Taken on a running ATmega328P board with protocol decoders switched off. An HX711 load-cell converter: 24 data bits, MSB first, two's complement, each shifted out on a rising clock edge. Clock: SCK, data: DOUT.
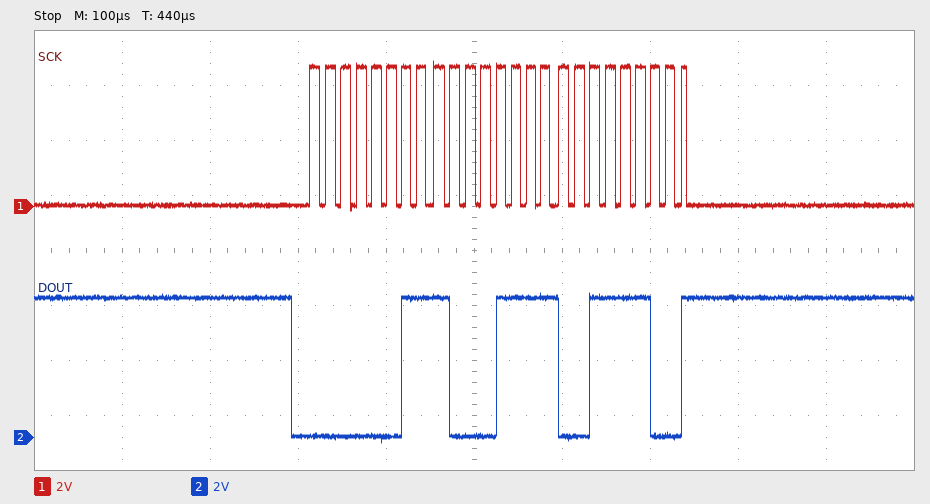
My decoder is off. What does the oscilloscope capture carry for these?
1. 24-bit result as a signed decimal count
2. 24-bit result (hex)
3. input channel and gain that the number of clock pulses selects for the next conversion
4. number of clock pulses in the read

233276
0x038F3C
channel A, gain 128
25
